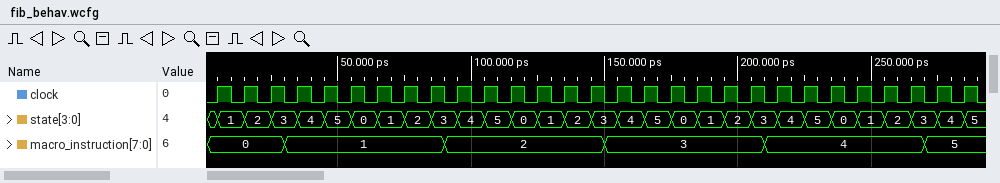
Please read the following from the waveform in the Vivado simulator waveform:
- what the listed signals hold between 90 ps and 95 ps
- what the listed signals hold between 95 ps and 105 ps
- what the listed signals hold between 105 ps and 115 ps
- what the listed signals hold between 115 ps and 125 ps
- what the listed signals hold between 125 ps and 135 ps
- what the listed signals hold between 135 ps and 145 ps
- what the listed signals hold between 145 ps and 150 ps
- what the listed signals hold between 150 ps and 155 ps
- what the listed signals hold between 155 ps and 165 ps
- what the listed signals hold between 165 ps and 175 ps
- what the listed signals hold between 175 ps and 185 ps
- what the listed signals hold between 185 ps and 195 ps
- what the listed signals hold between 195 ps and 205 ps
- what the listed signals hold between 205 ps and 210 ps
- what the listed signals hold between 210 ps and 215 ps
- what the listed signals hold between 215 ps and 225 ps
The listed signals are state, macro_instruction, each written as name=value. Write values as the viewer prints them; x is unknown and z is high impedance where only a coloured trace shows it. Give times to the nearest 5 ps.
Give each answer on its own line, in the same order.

state=3, macro_instruction=2
state=4, macro_instruction=2
state=5, macro_instruction=2
state=0, macro_instruction=2
state=1, macro_instruction=2
state=2, macro_instruction=2
state=3, macro_instruction=2
state=3, macro_instruction=3
state=4, macro_instruction=3
state=5, macro_instruction=3
state=0, macro_instruction=3
state=1, macro_instruction=3
state=2, macro_instruction=3
state=3, macro_instruction=3
state=3, macro_instruction=4
state=4, macro_instruction=4
